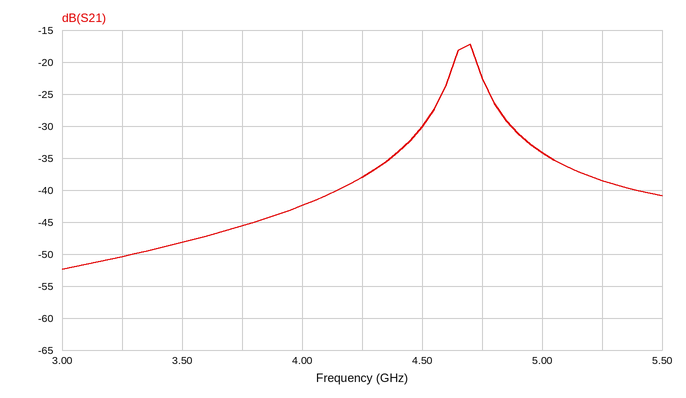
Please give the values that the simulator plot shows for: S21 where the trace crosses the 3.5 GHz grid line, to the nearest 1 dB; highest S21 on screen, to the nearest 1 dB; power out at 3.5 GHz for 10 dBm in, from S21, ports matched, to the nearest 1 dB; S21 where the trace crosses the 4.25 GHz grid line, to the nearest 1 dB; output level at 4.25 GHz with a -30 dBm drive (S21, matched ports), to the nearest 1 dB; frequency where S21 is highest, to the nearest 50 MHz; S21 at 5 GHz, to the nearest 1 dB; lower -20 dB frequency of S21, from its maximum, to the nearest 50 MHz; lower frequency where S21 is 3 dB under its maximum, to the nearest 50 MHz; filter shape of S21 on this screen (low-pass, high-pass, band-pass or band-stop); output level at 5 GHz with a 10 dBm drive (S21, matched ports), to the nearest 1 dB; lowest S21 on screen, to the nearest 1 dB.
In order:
-48 dB
-17 dB
-38 dBm
-38 dB
-68 dBm
4.70 GHz
-34 dB
4.30 GHz
4.65 GHz
band-pass
-24 dBm
-52 dB
